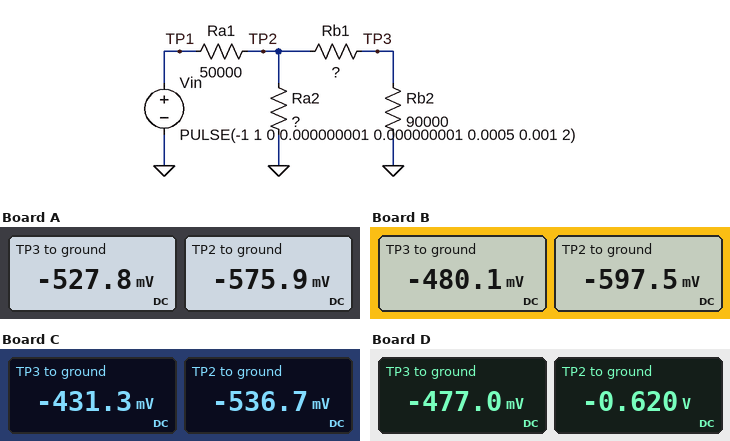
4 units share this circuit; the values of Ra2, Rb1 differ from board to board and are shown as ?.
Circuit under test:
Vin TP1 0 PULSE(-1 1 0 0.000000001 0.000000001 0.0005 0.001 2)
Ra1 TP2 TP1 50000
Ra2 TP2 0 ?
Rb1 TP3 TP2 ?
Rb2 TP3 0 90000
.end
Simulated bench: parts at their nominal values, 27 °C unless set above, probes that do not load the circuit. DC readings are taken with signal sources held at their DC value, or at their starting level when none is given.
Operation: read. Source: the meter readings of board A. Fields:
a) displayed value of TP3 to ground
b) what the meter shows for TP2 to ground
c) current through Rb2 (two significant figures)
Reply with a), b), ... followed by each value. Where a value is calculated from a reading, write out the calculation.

a) -527.8 mV
b) -575.9 mV
c) (0 V - (-527.8 mV)) / 90 kΩ = 5.9 µA
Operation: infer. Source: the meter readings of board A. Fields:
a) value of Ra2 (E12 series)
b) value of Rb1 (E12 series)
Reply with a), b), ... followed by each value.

a) 220 kΩ
b) 8.2 kΩ
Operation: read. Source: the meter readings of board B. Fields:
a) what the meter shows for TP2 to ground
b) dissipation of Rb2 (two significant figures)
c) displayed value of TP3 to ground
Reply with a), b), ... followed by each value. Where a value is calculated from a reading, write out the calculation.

a) -597.5 mV
b) (0 V - (-480.1 mV))^2 / 90 kΩ = 2.6 µW
c) -480.1 mV
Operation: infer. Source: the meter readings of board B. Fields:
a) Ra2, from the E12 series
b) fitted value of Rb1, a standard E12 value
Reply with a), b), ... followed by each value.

a) 220 kΩ
b) 22 kΩ
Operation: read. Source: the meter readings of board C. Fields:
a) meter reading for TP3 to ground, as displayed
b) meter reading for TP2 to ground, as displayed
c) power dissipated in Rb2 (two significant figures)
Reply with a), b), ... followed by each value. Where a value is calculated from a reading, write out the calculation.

a) -431.3 mV
b) -536.7 mV
c) (0 V - (-431.3 mV))^2 / 90 kΩ = 2.1 µW
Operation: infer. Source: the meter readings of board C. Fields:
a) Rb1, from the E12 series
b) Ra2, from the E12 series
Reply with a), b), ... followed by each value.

a) 22 kΩ
b) 120 kΩ
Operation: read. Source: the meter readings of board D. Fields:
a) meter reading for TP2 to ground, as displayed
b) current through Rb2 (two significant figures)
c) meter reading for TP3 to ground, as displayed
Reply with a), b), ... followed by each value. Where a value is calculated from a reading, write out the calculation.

a) -0.620 V
b) (0 V - (-477 mV)) / 90 kΩ = 5.3 µA
c) -477.0 mV
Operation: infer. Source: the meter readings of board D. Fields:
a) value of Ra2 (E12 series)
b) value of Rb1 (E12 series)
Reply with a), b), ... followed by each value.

a) 270 kΩ
b) 27 kΩ
